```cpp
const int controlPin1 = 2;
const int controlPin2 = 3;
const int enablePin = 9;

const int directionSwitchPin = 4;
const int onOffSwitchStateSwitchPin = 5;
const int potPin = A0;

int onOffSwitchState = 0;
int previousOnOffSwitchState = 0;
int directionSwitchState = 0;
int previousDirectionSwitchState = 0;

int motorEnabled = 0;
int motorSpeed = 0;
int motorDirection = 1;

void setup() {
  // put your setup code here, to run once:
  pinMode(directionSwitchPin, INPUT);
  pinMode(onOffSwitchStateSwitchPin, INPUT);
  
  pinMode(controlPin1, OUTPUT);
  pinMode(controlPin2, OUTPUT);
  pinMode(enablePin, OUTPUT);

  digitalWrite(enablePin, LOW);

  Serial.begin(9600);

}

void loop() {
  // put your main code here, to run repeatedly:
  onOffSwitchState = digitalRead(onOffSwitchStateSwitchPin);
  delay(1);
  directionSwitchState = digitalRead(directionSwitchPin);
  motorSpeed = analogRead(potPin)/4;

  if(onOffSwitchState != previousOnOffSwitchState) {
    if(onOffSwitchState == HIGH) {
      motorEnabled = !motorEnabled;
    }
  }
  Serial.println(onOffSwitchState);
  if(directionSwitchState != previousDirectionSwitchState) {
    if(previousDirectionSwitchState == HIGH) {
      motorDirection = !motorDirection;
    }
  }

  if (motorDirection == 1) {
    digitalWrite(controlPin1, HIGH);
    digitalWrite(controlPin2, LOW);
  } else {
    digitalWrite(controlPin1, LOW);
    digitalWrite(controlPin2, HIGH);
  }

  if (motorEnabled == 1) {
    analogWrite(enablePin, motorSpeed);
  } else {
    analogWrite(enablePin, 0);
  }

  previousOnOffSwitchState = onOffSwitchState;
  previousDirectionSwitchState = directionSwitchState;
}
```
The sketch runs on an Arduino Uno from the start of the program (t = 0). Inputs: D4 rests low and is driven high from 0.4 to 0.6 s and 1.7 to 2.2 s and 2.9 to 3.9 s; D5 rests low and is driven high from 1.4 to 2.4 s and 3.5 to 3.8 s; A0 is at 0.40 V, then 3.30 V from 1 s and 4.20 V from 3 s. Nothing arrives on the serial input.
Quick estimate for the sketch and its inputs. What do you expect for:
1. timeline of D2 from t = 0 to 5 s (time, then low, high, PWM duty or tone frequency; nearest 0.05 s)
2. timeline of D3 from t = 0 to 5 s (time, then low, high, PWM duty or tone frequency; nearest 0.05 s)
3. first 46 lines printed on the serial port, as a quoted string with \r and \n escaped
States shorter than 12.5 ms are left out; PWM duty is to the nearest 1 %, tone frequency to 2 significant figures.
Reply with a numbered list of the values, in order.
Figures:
1. 0 s high; 0.6 s low; 2.2 s high; 3.9 s low
2. 0 s low; 0.6 s high; 2.2 s low; 3.9 s high
3. "0\r\n0\r\n0\r\n0\r\n0\r\n0\r\n0\r\n0\r\n0\r\n0\r\n0\r\n0\r\n0\r\n0\r\n0\r\n0\r\n0\r\n0\r\n0\r\n0\r\n0\r\n0\r\n0\r\n0\r\n0\r\n0\r\n0\r\n0\r\n0\r\n0\r\n0\r\n0\r\n0\r\n0\r\n0\r\n0\r\n0\r\n0\r\n0\r\n0\r\n0\r\n0\r\n0\r\n0\r\n0\r\n0\r\n"
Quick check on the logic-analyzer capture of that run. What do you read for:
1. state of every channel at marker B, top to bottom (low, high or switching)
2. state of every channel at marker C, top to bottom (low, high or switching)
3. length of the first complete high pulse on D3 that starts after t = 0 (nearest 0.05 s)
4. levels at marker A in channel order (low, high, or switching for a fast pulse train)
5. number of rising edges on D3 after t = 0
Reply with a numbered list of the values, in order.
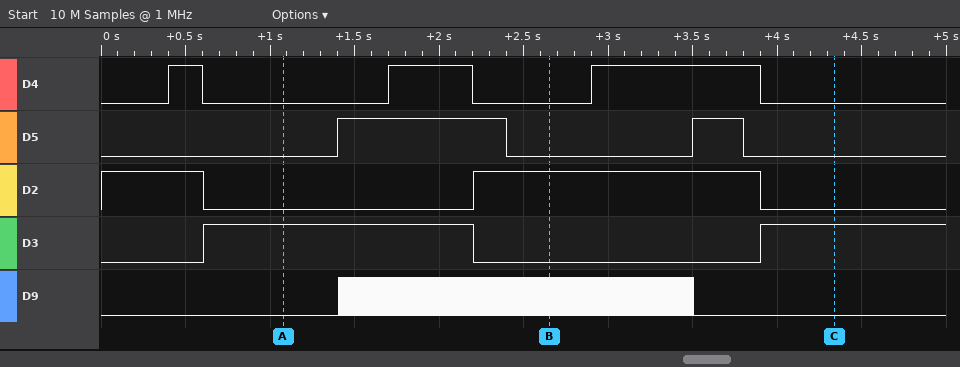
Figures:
1. D4 low, D5 low, D2 high, D3 low, D9 switching
2. D4 low, D5 low, D2 low, D3 high, D9 low
3. 1.60 s
4. D4 low, D5 low, D2 low, D3 high, D9 low
5. 2
